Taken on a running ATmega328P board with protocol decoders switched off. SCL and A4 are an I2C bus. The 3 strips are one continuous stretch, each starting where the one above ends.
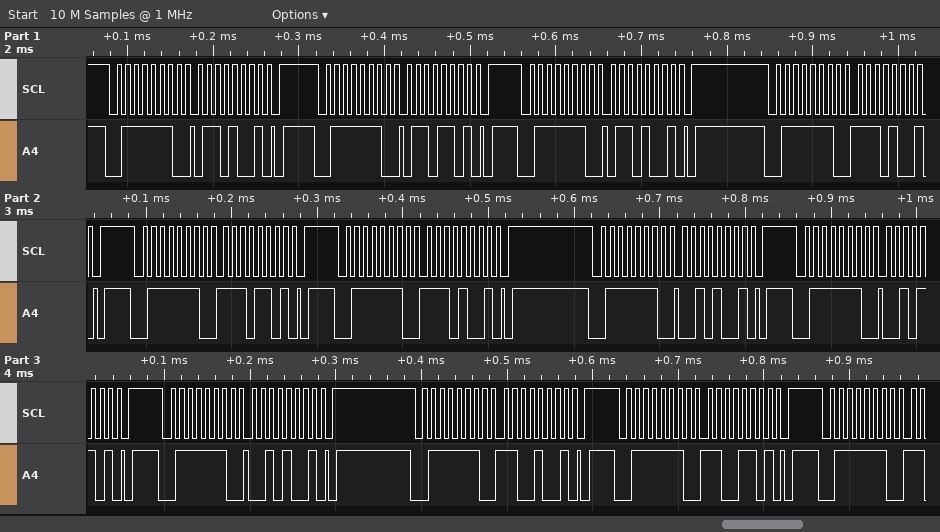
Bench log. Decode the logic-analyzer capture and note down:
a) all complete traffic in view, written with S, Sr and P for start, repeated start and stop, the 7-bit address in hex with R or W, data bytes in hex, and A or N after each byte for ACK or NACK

S 3FW A 69 A P S 3FW A 6D A P S 3FW A 69 A P S 3FW A E9 A P S 3FW A ED A P S 3FW A E9 A P S 3FW A 29 A P S 3FW A 2D A P S 3FW A 29 A P S 3FW A C9 A P S 3FW A CD A P S 3FW A
